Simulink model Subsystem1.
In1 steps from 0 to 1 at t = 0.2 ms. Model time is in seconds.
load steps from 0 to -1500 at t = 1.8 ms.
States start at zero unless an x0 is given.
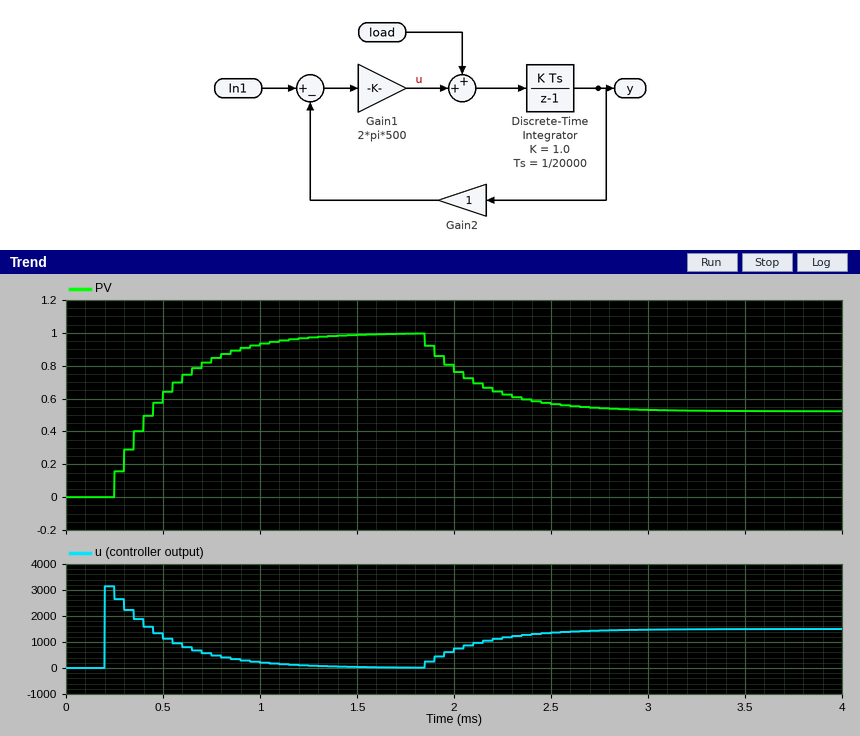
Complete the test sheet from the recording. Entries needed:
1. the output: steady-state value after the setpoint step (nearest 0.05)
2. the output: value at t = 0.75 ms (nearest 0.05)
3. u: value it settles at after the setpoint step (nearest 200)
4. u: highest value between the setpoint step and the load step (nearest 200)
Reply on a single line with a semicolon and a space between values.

1.00; 0.85; 0; 3200
